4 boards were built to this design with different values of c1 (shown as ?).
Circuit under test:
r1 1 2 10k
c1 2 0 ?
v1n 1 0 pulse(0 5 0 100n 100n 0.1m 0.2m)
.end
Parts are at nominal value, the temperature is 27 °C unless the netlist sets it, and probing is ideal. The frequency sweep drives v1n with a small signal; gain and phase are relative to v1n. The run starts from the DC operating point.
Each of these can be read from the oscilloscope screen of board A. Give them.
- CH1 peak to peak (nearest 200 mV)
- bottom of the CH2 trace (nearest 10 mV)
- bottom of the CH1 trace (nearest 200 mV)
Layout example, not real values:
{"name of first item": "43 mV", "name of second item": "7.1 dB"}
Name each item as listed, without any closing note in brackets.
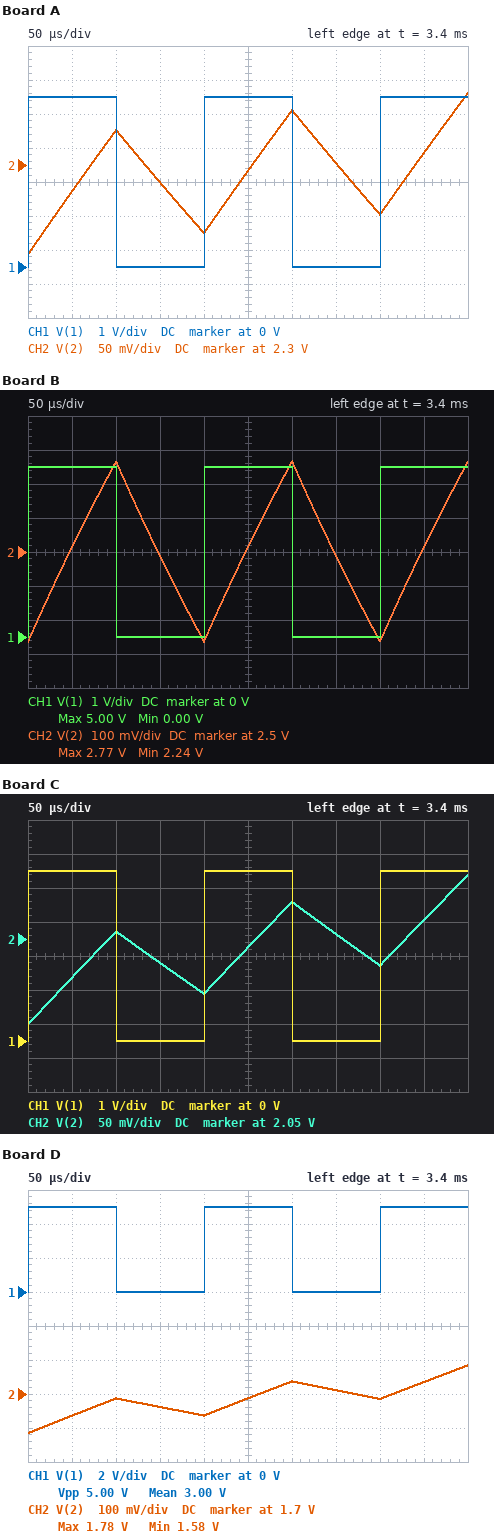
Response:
{"CH1 peak to peak": "5.0 V", "bottom of the CH2 trace": "2.17 V", "bottom of the CH1 trace": "0 V"}
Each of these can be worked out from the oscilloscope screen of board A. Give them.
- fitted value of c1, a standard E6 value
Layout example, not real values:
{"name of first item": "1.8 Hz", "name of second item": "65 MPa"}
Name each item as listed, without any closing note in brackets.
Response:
{"fitted value of c1, a standard E6 value": "150 nF"}
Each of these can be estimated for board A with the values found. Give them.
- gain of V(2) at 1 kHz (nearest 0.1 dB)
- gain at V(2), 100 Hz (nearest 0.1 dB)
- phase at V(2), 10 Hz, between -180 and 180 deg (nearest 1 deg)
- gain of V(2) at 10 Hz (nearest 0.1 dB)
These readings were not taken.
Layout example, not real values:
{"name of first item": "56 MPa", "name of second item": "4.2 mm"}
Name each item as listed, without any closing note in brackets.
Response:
{"gain of V(2) at 1 kHz": "-19.5 dB", "gain at V(2), 100 Hz": "-2.8 dB", "phase at V(2), 10 Hz, between -180 and 180 deg": "-5 deg", "gain of V(2) at 10 Hz": "0 dB"}
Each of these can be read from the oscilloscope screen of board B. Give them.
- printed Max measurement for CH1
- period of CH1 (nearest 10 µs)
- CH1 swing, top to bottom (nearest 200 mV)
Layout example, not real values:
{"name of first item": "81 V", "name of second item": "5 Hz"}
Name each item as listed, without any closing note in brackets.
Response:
{"printed Max measurement for CH1": "5.00 V", "period of CH1": "200 µs", "CH1 swing, top to bottom": "5.0 V"}
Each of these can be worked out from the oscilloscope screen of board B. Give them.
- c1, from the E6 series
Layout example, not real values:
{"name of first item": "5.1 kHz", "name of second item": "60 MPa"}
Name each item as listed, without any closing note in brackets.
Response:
{"c1, from the E6 series": "47 nF"}
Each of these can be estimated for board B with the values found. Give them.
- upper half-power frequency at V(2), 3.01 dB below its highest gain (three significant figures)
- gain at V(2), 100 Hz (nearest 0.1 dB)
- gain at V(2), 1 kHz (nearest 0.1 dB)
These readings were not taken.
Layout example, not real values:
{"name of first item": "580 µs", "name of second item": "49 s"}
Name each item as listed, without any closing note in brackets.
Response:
{"upper half-power frequency at V(2), 3.01 dB below its highest gain": "339 Hz", "gain at V(2), 100 Hz": "-0.4 dB", "gain at V(2), 1 kHz": "-9.9 dB"}
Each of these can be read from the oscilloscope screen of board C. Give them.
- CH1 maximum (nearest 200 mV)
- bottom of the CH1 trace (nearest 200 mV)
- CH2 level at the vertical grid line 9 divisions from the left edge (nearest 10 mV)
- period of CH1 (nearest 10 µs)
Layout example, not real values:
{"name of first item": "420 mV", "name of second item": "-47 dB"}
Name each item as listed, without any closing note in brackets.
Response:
{"CH1 maximum": "5.0 V", "bottom of the CH1 trace": "0 V", "CH2 level at the vertical grid line 9 divisions from the left edge": "2.08 V", "period of CH1": "200 µs"}
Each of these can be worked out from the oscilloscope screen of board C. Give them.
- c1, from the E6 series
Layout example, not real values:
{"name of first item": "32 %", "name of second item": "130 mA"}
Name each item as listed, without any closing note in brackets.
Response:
{"c1, from the E6 series": "220 nF"}
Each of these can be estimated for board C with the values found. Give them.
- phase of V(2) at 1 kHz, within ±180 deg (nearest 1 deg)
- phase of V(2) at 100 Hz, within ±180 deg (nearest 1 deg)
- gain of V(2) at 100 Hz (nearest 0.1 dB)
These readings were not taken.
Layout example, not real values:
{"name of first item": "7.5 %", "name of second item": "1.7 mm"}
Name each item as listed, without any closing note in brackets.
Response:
{"phase of V(2) at 1 kHz, within ±180 deg": "-86 deg", "phase of V(2) at 100 Hz, within ±180 deg": "-54 deg", "gain of V(2) at 100 Hz": "-4.6 dB"}
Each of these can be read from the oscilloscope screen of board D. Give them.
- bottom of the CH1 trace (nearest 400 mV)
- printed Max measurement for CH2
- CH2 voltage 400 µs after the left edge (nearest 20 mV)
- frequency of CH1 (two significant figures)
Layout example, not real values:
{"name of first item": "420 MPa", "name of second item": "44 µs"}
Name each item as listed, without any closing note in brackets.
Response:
{"bottom of the CH1 trace": "0 V", "printed Max measurement for CH2": "1.78 V", "CH2 voltage 400 µs after the left edge": "1.68 V", "frequency of CH1": "5.0 kHz"}
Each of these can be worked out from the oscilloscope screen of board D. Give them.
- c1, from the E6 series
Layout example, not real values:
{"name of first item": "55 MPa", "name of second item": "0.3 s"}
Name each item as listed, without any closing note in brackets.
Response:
{"c1, from the E6 series": "330 nF"}
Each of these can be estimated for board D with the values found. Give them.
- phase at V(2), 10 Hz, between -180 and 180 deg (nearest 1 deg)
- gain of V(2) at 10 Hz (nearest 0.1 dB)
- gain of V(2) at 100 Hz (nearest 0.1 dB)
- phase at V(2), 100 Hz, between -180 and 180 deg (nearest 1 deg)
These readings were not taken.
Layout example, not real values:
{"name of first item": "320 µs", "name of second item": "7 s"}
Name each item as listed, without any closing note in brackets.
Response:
{"phase at V(2), 10 Hz, between -180 and 180 deg": "-12 deg", "gain of V(2) at 10 Hz": "-0.2 dB", "gain of V(2) at 100 Hz": "-7.2 dB", "phase at V(2), 100 Hz, between -180 and 180 deg": "-64 deg"}
